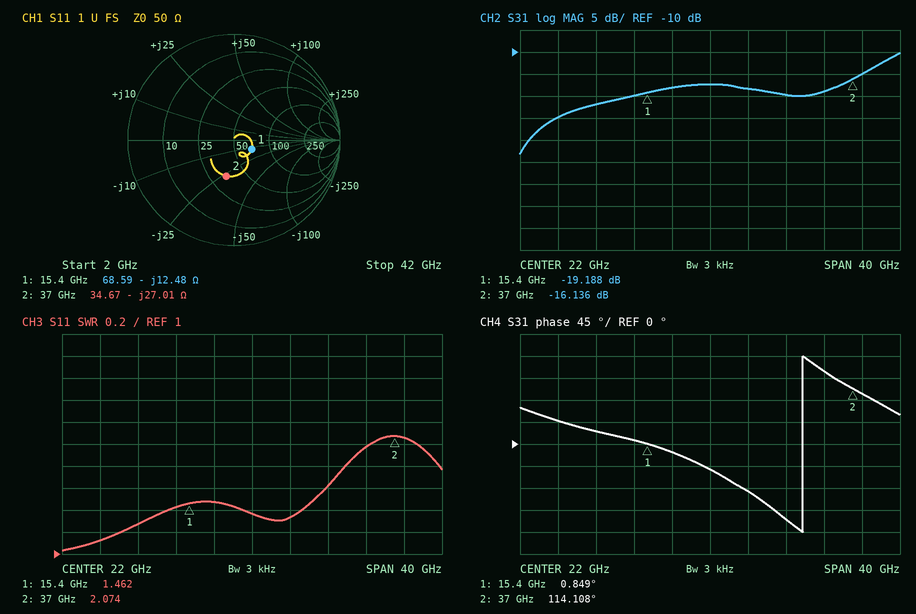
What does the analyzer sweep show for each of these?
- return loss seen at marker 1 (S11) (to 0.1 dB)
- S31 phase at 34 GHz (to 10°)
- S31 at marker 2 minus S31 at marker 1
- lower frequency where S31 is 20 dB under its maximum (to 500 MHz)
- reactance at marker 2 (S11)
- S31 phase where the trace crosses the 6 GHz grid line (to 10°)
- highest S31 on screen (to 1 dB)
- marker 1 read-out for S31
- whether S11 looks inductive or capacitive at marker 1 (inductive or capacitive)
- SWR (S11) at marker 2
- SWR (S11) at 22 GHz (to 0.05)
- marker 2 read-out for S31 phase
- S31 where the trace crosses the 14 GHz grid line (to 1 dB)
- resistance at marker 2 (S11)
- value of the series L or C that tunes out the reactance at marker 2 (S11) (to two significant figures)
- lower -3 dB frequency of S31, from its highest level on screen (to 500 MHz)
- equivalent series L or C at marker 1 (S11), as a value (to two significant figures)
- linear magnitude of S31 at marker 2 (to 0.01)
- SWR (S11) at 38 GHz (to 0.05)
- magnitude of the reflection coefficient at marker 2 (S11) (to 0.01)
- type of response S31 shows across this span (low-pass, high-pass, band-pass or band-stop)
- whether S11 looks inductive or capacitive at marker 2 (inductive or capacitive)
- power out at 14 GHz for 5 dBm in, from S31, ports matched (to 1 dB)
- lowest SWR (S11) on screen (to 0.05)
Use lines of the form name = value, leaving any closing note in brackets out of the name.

return loss seen at marker 1 (S11) = 14.5 dB
S31 phase at 34 GHz = 150°
S31 at marker 2 minus S31 at marker 1 = 3.052 dB
lower frequency where S31 is 20 dB under its maximum = 3.0 GHz
reactance at marker 2 = -27.01 Ω
S31 phase where the trace crosses the 6 GHz grid line = 50°
highest S31 on screen = -10 dB
marker 1 read-out for S31 = -19.188 dB
whether S11 looks inductive or capacitive at marker 1 = capacitive
SWR (S11) at marker 2 = 2.074
SWR (S11) at 22 GHz = 1.35
marker 2 read-out for S31 phase = 114.108°
S31 where the trace crosses the 14 GHz grid line = -20 dB
resistance at marker 2 = 34.67 Ω
value of the series L or C that tunes out the reactance at marker 2 (S11) = 120 pH
lower -3 dB frequency of S31, from its highest level on screen = 39.5 GHz
equivalent series L or C at marker 1 (S11), as a value = 830 fF
linear magnitude of S31 at marker 2 = 0.16
SWR (S11) at 38 GHz = 2.05
magnitude of the reflection coefficient at marker 2 (S11) = 0.35
type of response S31 shows across this span = high-pass
whether S11 looks inductive or capacitive at marker 2 = capacitive
power out at 14 GHz for 5 dBm in, from S31, ports matched = -15 dBm
lowest SWR (S11) on screen = 1.05
